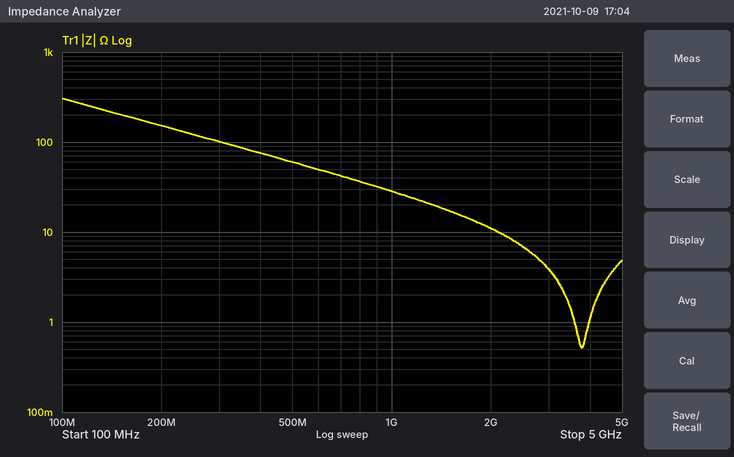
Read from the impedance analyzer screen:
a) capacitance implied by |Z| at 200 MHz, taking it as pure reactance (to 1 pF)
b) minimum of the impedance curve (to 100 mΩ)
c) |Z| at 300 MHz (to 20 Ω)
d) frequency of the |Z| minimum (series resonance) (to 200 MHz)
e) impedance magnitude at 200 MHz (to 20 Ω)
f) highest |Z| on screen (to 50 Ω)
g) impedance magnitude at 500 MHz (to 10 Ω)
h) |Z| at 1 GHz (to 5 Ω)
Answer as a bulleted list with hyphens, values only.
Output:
- 5 pF
- 500 mΩ
- 100 Ω
- 3.8 GHz
- 160 Ω
- 300 Ω
- 60 Ω
- 30 Ω
